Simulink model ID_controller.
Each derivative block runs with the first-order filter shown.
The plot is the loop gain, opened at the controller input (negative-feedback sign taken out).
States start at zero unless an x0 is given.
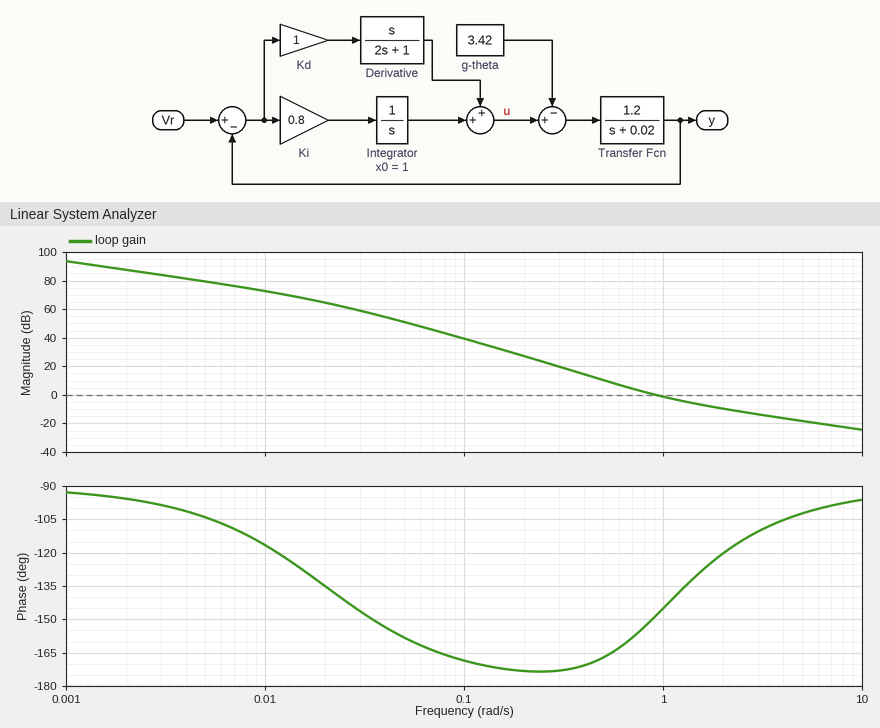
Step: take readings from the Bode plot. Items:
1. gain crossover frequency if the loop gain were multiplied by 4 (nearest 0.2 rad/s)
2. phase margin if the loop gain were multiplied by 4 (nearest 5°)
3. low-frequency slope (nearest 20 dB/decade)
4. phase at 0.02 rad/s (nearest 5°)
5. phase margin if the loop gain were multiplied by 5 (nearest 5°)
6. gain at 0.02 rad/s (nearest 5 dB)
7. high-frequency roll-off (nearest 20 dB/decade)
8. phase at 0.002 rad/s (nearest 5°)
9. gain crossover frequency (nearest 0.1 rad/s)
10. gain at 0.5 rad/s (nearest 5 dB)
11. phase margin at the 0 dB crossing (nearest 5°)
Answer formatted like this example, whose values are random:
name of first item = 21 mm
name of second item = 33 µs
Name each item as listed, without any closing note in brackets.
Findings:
gain crossover frequency if the loop gain were multiplied by 4 = 2.6 rad/s
phase margin if the loop gain were multiplied by 4 = 65°
low-frequency slope = -20 dB/decade
phase at 0.02 rad/s = -135°
phase margin if the loop gain were multiplied by 5 = 70°
gain at 0.02 rad/s = 65 dB
high-frequency roll-off = -20 dB/decade
phase at 0.002 rad/s = -95°
gain crossover frequency = 0.9 rad/s
gain at 0.5 rad/s = 10 dB
phase margin at the 0 dB crossing = 30°
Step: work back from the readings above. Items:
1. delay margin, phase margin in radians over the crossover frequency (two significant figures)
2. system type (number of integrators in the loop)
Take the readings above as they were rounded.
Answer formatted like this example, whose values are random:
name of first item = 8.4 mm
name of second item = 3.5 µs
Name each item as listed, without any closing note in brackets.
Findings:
delay margin, phase margin in radians over the crossover frequency = 0.58 s
system type = 1
